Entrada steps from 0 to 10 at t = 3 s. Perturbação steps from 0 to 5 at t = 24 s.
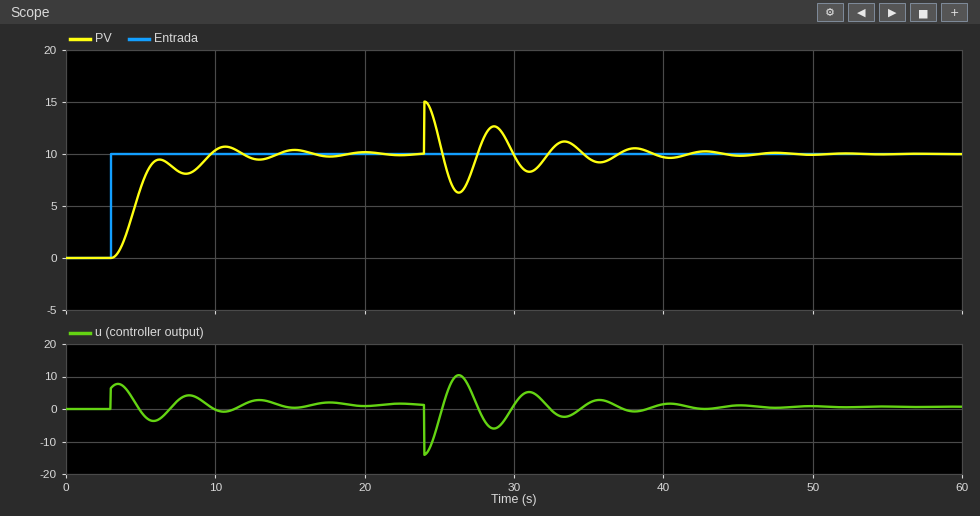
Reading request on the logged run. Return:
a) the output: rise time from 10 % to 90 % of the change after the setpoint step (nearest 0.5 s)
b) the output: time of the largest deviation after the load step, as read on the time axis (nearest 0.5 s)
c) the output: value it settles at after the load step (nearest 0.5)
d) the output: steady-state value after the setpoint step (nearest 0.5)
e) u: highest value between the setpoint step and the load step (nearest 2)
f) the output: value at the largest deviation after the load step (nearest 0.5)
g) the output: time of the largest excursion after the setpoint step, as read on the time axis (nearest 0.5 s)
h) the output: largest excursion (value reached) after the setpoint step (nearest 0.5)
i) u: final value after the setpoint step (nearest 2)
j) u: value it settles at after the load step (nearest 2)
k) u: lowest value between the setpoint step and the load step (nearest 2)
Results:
2.0 s
24.0 s
10.0
10.0
8
15.0
10.5 s
10.5
2
0
-4
